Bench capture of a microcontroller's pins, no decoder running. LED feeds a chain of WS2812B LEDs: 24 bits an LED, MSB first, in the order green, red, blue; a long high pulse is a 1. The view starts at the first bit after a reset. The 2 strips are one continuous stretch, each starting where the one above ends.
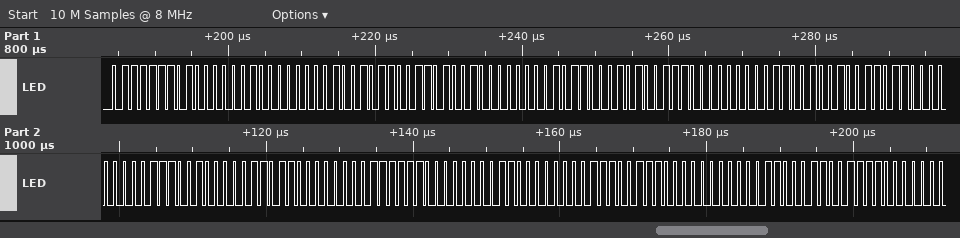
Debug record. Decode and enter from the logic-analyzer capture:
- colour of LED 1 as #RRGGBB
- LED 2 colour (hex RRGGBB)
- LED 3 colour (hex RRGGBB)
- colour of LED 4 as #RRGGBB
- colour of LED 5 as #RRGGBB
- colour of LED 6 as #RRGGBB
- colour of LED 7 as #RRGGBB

#817E00
#699600
#4EB100
#36C900
#1BE400
#03FC00
#00E718
